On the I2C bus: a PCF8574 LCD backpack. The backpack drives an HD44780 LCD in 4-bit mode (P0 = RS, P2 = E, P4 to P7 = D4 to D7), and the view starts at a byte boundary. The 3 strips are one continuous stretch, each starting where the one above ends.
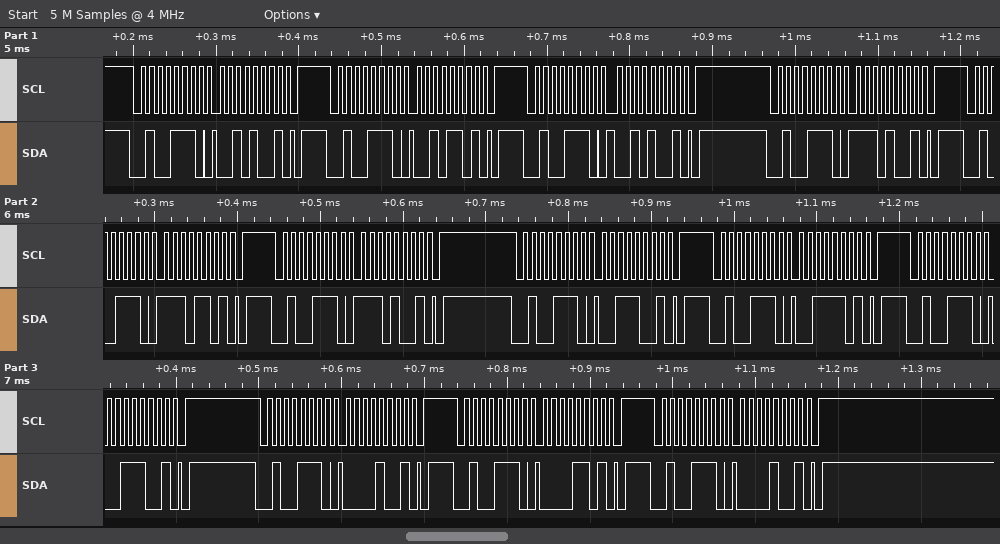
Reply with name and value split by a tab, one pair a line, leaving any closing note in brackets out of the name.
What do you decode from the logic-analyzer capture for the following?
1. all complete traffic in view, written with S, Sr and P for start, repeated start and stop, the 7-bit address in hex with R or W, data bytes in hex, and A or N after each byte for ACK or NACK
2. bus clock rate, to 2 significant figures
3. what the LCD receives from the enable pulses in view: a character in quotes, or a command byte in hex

all complete traffic in view, written with S, Sr and P for start, repeated start and stop, the 7-bit address in hex with R or W, data bytes in hex, and A or N after each byte for ACK or NACK	S 27W A 29 A P S 27W A 2D A P S 27W A 29 A P S 27W A E9 A P S 27W A ED A P S 27W A E9 A P S 27W A 39 A P S 27W A 3D A P S 27W A 39 A P S 27W A 09 A P S 27W A 0D A P S 27W A 09 A P
bus clock rate, to 2 significant figures	100 kHz
what the LCD receives from the enable pulses in view: a character in quotes, or a command byte in hex	'.' '0'
